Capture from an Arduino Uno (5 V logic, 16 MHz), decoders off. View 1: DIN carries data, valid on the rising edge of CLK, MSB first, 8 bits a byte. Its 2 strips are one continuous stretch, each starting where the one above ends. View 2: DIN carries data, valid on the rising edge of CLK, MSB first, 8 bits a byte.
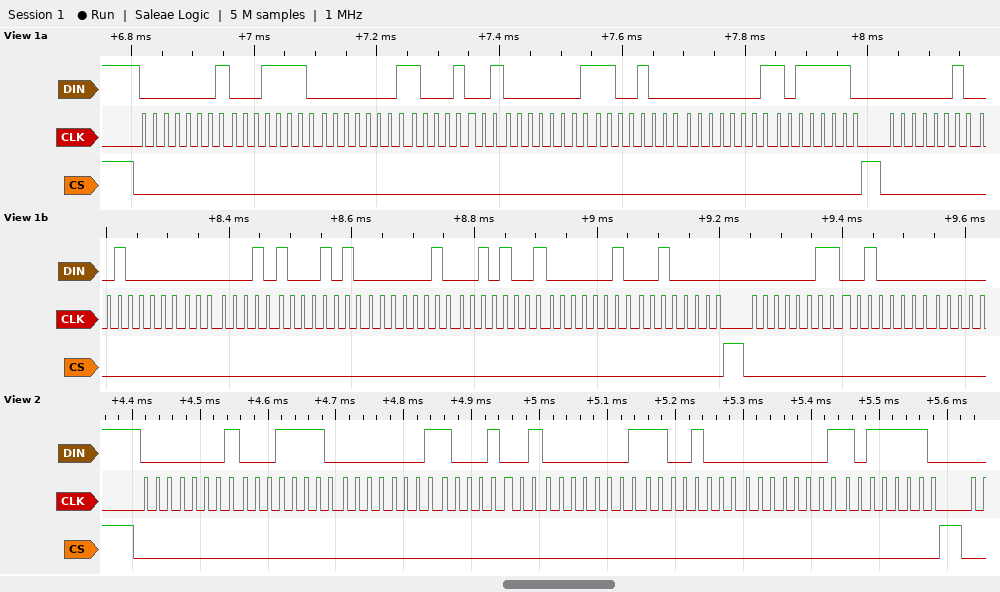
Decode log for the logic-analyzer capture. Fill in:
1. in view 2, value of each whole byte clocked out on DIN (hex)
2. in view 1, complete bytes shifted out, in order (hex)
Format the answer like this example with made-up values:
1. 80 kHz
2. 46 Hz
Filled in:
1. 01 1E 01 89 01 C8 01 BE
2. 0x01 0x1E 0x01 0x89 0x01 0xC8 0x01 0xBE 0x02 0x20 0x02 0x8A 0x02 0x29 0x02 0x20 0x03 0x20
